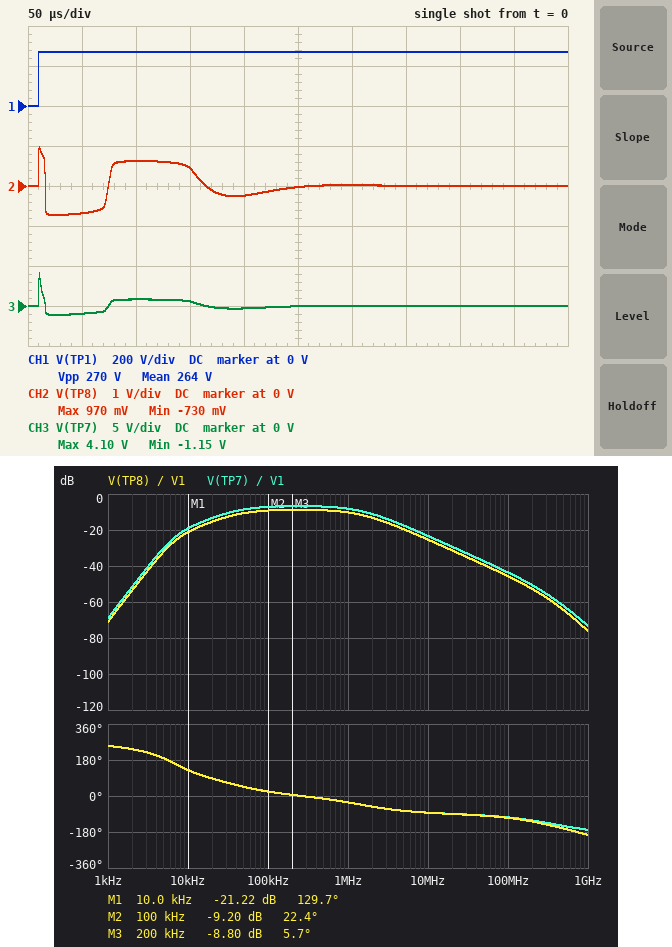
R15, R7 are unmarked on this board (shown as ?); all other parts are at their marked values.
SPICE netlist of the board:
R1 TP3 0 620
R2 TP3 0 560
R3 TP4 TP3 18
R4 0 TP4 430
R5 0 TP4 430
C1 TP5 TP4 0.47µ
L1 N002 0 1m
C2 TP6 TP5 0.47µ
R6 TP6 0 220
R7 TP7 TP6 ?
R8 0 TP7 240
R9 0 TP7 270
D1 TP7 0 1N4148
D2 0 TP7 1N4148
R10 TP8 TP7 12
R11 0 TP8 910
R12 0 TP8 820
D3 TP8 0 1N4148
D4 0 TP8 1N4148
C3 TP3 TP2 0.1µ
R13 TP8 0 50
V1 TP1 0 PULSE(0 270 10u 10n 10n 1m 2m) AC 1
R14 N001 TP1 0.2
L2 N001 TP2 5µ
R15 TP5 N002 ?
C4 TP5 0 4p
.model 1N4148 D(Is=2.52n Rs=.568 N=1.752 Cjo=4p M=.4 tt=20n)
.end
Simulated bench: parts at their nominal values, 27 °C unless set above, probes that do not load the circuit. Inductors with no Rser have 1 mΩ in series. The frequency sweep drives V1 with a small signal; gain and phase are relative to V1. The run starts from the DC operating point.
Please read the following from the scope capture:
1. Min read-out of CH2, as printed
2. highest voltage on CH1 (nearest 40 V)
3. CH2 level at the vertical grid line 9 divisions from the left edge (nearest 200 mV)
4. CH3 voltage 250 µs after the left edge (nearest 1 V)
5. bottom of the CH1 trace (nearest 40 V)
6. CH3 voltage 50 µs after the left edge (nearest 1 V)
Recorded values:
-730 mV
280 V
0 V
0 V
0 V
-1 V
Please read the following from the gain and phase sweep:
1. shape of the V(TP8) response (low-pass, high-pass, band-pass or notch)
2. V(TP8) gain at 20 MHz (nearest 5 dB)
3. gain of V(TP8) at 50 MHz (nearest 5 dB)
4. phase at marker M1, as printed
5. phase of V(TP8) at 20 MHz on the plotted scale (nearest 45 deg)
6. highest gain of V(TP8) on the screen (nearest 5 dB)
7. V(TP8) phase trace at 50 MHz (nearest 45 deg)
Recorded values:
band-pass
-30 dB
-40 dB
129.7 deg
-90 deg
-10 dB
-90 deg
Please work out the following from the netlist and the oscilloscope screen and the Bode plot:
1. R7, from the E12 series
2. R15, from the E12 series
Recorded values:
18 Ω
18 Ω
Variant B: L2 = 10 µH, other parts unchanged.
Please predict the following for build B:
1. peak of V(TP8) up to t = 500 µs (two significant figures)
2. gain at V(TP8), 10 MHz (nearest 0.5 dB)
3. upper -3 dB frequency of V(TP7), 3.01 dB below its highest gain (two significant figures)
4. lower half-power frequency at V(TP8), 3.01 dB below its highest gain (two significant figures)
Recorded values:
950 mV
-31.5 dB
780 kHz
36 kHz
